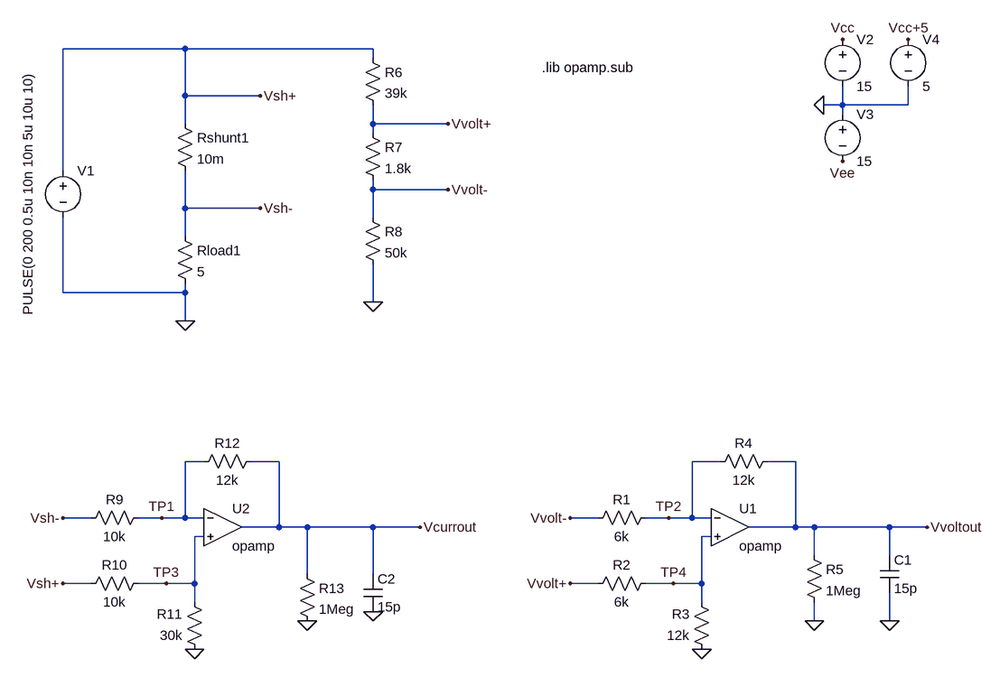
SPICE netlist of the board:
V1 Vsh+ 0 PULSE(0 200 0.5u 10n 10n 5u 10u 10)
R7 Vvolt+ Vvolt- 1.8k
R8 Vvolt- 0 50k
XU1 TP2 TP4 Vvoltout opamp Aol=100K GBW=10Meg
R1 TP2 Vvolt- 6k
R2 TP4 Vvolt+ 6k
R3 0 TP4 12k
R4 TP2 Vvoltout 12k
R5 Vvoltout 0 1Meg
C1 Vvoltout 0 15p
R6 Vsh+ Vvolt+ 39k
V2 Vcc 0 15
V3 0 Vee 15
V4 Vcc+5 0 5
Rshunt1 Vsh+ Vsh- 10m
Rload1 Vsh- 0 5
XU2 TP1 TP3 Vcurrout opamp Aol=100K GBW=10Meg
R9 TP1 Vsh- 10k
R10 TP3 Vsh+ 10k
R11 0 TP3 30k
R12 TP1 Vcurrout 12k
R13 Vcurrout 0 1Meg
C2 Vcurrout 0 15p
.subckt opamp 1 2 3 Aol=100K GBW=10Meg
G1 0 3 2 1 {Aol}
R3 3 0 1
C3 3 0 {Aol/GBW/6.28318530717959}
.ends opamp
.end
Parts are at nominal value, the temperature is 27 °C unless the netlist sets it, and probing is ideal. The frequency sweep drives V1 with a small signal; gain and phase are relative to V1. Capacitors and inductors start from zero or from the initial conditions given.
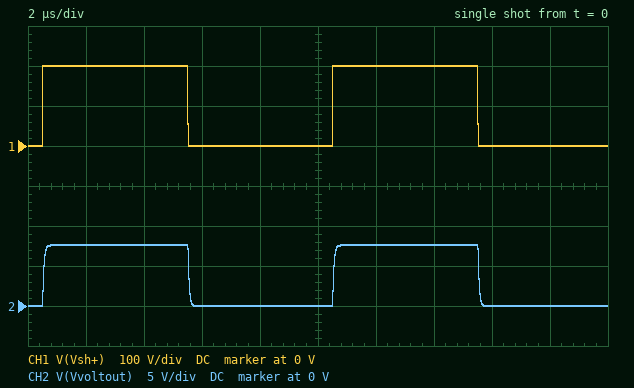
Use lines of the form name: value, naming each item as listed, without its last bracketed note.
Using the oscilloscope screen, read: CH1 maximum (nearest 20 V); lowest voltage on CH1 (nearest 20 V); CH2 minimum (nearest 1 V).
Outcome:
CH1 maximum: 200 V
lowest voltage on CH1: 0 V
CH2 minimum: 0 V
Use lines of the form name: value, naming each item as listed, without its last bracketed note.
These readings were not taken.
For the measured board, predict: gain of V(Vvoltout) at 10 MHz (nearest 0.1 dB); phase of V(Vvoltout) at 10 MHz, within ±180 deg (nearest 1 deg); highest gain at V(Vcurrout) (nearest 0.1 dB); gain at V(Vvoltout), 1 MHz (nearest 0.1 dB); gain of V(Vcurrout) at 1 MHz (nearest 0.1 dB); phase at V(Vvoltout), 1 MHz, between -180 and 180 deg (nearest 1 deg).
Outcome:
gain of V(Vvoltout) at 10 MHz: -37.7 dB
phase of V(Vvoltout) at 10 MHz, within ±180 deg: -70 deg
highest gain at V(Vcurrout): -6.9 dB
gain at V(Vvoltout), 1 MHz: -28.7 dB
gain of V(Vcurrout) at 1 MHz: -7.1 dB
phase at V(Vvoltout), 1 MHz, between -180 and 180 deg: -15 deg
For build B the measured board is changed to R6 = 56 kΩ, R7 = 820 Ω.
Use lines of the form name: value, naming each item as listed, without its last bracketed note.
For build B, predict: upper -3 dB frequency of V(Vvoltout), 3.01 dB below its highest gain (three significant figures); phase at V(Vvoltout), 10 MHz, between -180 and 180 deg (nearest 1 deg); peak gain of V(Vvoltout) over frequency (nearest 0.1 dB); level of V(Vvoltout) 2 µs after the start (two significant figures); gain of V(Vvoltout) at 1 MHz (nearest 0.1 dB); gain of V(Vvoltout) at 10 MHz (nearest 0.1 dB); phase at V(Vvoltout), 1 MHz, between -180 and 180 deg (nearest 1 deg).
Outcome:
upper -3 dB frequency of V(Vvoltout), 3.01 dB below its highest gain: 3.48 MHz
phase at V(Vvoltout), 10 MHz, between -180 and 180 deg: -71 deg
peak gain of V(Vvoltout) over frequency: -37.2 dB
level of V(Vvoltout) 2 µs after the start: 2.8 V
gain of V(Vvoltout) at 1 MHz: -37.5 dB
gain of V(Vvoltout) at 10 MHz: -46.9 dB
phase at V(Vvoltout), 1 MHz, between -180 and 180 deg: -16 deg
